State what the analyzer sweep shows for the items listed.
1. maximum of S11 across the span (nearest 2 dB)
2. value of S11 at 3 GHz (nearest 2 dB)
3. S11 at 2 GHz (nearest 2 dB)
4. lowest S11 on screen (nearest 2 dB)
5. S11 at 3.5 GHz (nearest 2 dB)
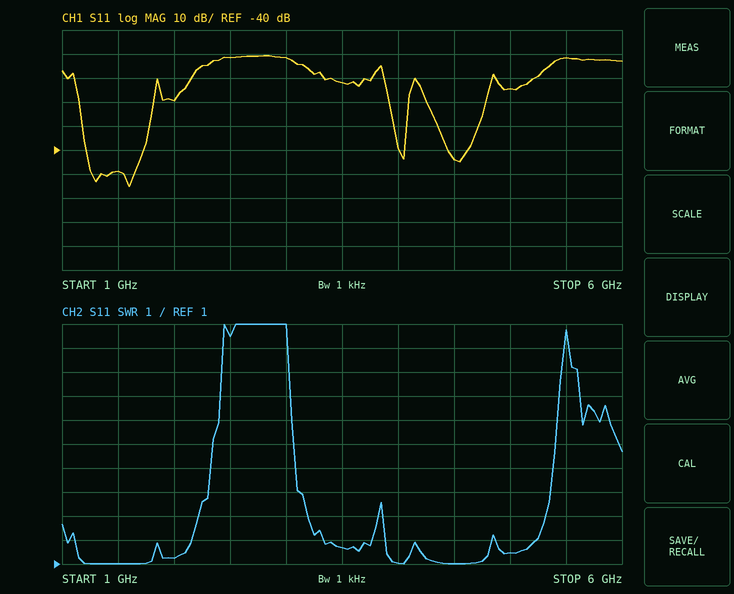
0 dB
-2 dB
-20 dB
-56 dB
-12 dB
